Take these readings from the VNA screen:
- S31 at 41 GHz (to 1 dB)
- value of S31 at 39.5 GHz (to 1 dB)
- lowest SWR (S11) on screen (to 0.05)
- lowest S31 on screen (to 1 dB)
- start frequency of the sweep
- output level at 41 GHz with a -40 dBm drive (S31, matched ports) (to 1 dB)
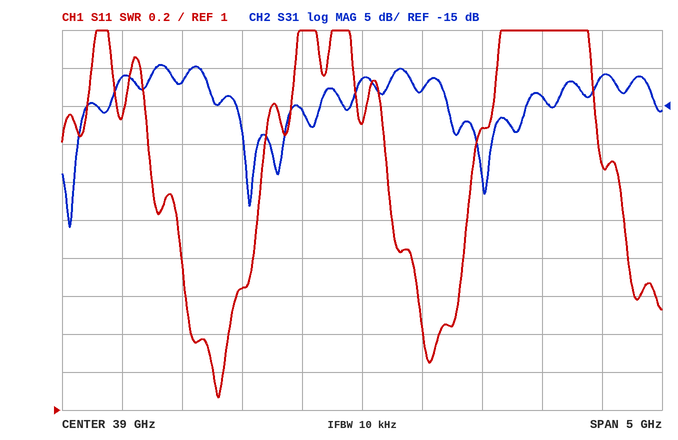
-11 dB
-13 dB
1.05
-31 dB
36.5 GHz
-51 dBm
